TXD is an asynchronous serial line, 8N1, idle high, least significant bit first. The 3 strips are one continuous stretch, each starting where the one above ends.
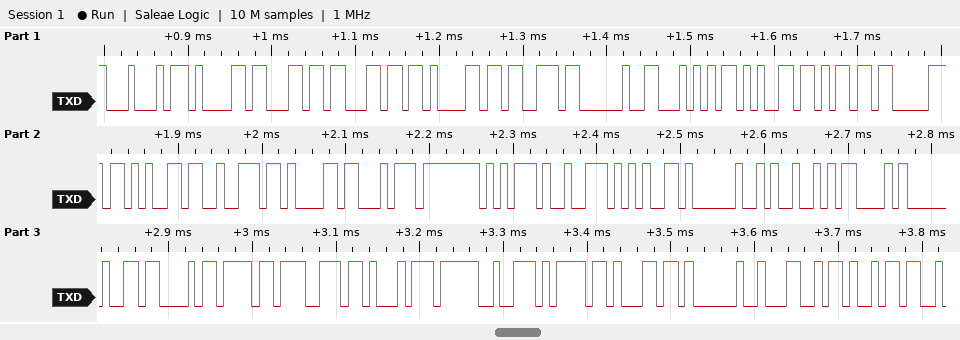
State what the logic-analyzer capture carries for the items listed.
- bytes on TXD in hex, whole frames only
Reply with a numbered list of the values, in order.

1. 44 61 6C 6C 61 73 20 54 65 6D 70 65 72 61 74 75 72 65 20 49 43 20 43 6F 6E 74 72 6F 6C 20 4C 69
